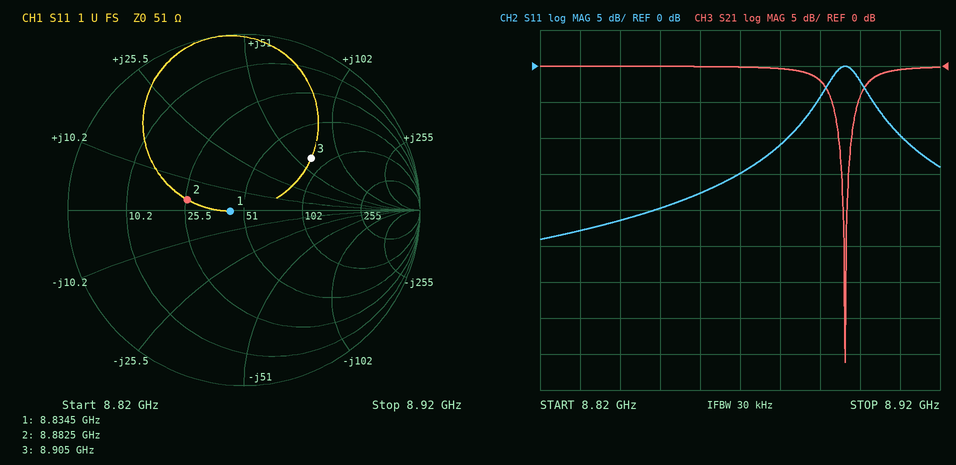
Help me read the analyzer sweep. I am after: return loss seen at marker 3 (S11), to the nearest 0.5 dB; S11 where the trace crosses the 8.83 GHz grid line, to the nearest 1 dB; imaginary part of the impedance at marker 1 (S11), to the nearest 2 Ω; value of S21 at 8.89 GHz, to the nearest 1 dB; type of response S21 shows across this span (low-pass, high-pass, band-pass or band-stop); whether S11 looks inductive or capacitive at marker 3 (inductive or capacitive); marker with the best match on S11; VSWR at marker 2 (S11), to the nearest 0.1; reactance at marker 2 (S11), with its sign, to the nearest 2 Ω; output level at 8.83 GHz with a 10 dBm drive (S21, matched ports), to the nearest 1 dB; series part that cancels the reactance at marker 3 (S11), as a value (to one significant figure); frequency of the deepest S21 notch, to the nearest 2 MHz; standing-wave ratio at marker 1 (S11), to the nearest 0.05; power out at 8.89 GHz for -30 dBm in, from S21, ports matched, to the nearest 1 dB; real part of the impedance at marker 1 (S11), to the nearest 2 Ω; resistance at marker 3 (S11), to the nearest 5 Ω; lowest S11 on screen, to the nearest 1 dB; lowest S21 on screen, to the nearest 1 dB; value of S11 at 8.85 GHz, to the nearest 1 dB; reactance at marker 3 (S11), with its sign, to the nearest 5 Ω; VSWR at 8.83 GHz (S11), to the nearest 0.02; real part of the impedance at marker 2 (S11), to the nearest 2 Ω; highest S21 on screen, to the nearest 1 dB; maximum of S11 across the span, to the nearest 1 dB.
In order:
6.5 dB
-23 dB
0 Ω
-2 dB
band-stop
inductive
marker 1
2.0
+4 Ω
10 dBm
300 fF
8.896 GHz
1.15
-32 dBm
44 Ω
85 Ω
-24 dB
-41 dB
-20 dB
+65 Ω
1.16
26 Ω
0 dB
0 dB
